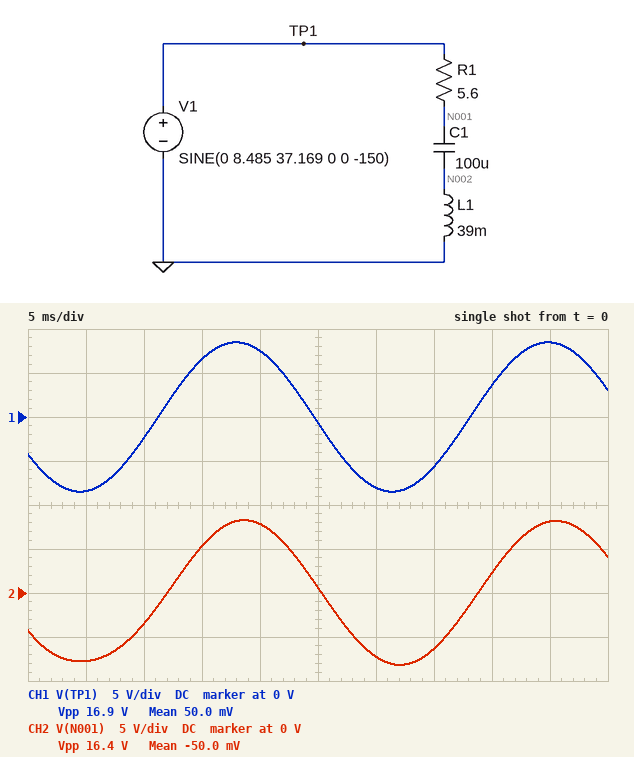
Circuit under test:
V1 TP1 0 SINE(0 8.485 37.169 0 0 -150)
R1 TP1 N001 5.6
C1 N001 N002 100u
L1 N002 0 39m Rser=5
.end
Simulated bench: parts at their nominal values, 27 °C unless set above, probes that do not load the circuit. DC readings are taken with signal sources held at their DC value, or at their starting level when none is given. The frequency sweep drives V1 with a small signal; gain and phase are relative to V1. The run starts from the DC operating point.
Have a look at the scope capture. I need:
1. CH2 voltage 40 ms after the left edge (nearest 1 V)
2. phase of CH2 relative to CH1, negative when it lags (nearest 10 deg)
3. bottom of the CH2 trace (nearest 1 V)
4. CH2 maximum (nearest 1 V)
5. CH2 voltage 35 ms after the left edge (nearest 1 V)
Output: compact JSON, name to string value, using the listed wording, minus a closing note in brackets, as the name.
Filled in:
{"CH2 voltage 40 ms after the left edge": "2 V", "phase of CH2 relative to CH1, negative when it lags": "-10 deg", "bottom of the CH2 trace": "-8 V", "CH2 maximum": "8 V", "CH2 voltage 35 ms after the left edge": "-6 V"}
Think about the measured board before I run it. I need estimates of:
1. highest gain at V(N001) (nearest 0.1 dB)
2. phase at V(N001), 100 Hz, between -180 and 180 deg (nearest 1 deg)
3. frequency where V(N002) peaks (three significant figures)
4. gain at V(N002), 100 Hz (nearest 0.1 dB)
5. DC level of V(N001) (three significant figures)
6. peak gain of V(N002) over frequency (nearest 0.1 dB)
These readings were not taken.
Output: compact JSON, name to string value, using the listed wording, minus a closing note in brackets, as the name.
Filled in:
{"highest gain at V(N001)": "0 dB", "phase at V(N001), 100 Hz, between -180 and 180 deg": "21 deg", "frequency where V(N002) peaks": "86.7 Hz", "gain at V(N002), 100 Hz": "5.3 dB", "DC level of V(N001)": "-4.24 V", "peak gain of V(N002) over frequency": "6.0 dB"}
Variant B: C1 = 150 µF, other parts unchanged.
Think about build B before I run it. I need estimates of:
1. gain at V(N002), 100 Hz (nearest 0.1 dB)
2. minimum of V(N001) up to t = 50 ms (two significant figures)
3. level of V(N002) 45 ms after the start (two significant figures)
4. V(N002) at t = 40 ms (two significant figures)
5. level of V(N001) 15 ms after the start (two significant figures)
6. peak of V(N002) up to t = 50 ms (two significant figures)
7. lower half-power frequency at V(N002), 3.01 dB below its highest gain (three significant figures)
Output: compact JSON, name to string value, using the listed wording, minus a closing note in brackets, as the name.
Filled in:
{"gain at V(N002), 100 Hz": "3.1 dB", "minimum of V(N001) up to t = 50 ms": "-7.7 V", "level of V(N002) 45 ms after the start": "-2.3 V", "V(N002) at t = 40 ms": "2.1 V", "level of V(N001) 15 ms after the start": "4.4 V", "peak of V(N002) up to t = 50 ms": "4.6 V", "lower half-power frequency at V(N002), 3.01 dB below its highest gain": "54.8 Hz"}
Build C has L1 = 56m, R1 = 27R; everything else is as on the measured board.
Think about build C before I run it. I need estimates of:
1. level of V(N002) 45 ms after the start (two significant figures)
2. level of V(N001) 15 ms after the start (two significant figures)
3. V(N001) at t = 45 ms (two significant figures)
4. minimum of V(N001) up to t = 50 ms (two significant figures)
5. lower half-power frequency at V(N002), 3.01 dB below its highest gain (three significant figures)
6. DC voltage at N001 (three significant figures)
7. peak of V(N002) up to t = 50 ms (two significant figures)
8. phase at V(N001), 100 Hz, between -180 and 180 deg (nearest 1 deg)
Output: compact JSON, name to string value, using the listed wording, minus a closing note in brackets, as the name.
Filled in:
{"level of V(N002) 45 ms after the start": "-1.1 V", "level of V(N001) 15 ms after the start": "1.4 V", "V(N001) at t = 45 ms": "4.8 V", "minimum of V(N001) up to t = 50 ms": "-6.5 V", "lower half-power frequency at V(N002), 3.01 dB below its highest gain": "63.4 Hz", "DC voltage at N001": "-4.24 V", "peak of V(N002) up to t = 50 ms": "2.7 V", "phase at V(N001), 100 Hz, between -180 and 180 deg": "44 deg"}
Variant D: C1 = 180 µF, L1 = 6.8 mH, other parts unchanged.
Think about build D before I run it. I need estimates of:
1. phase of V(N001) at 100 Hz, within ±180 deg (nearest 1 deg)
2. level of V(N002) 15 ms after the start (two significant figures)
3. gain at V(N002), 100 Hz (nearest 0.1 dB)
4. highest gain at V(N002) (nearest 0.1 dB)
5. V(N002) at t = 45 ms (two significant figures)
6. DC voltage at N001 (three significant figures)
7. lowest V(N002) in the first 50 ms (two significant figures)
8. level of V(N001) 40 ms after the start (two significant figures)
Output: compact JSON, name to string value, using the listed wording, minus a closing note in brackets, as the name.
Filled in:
{"phase of V(N001) at 100 Hz, within ±180 deg": "-19 deg", "level of V(N002) 15 ms after the start": "1.3 V", "gain at V(N002), 100 Hz": "-4.9 dB", "highest gain at V(N002)": "0 dB", "V(N002) at t = 45 ms": "180 mV", "DC voltage at N001": "-4.24 V", "lowest V(N002) in the first 50 ms": "-1.8 V", "level of V(N001) 40 ms after the start": "1.7 V"}
